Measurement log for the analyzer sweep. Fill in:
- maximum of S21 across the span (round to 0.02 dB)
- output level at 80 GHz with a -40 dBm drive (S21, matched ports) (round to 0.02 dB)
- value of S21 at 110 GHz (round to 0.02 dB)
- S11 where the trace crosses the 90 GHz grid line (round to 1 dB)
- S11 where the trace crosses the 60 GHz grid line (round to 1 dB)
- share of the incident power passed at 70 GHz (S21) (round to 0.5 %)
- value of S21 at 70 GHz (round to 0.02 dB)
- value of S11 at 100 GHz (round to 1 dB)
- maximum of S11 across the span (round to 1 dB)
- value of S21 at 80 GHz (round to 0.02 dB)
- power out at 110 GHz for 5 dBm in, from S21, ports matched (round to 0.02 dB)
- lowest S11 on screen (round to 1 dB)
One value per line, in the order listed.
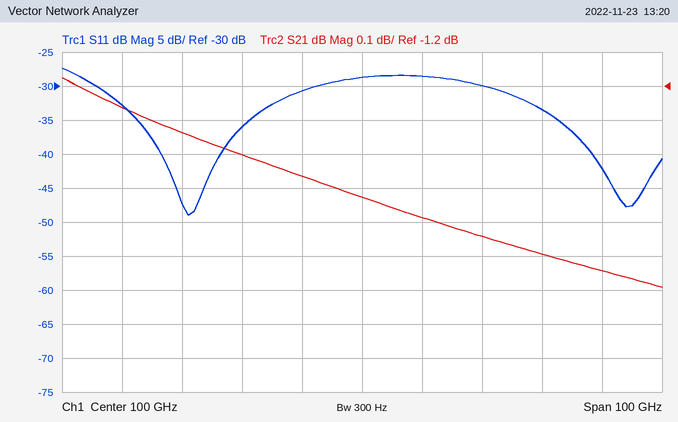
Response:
-1.18 dB
-41.40 dBm
-1.58 dB
-31 dB
-33 dB
73.5 %
-1.34 dB
-29 dB
-27 dB
-1.40 dB
3.42 dBm
-49 dB
